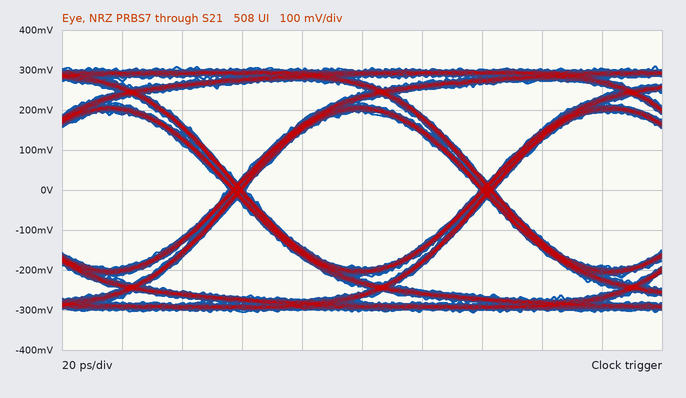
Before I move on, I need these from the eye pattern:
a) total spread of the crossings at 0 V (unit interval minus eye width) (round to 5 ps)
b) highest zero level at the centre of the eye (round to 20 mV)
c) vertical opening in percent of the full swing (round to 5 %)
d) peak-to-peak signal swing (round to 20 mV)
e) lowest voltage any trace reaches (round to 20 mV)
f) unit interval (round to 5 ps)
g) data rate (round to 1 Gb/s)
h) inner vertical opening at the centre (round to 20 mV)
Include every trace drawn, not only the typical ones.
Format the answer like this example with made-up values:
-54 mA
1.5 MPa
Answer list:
5 ps
-200 mV
65 %
620 mV
-300 mV
85 ps
12 Gb/s
400 mV
